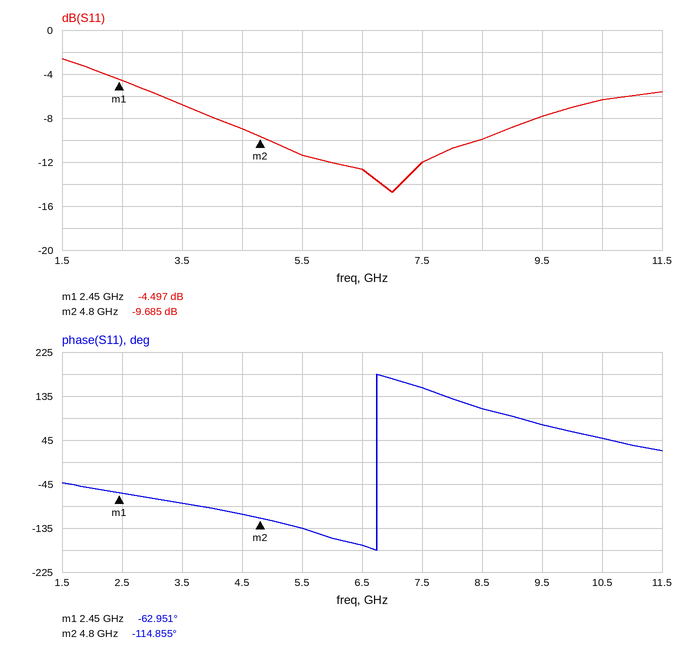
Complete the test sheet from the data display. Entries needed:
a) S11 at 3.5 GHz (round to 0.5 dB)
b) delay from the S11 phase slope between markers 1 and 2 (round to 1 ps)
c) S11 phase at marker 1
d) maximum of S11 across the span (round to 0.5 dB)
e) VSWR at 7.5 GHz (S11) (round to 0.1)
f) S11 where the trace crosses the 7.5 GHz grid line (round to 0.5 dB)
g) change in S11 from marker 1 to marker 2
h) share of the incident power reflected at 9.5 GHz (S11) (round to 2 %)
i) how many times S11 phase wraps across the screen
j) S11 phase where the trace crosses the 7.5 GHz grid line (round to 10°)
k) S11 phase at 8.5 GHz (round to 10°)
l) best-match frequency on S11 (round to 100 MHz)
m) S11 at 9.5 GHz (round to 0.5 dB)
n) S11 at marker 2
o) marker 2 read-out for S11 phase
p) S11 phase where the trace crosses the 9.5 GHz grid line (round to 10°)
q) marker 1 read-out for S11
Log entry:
-7.0 dB
61 ps
-62.951°
-2.5 dB
1.7
-12.0 dB
-5.188 dB
16 %
1
150°
110°
7.0 GHz
-8.0 dB
-9.685 dB
-114.855°
80°
-4.497 dB
